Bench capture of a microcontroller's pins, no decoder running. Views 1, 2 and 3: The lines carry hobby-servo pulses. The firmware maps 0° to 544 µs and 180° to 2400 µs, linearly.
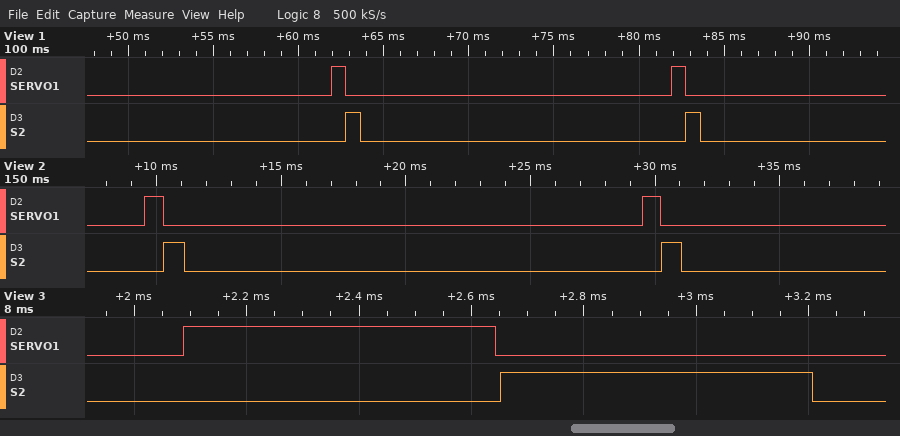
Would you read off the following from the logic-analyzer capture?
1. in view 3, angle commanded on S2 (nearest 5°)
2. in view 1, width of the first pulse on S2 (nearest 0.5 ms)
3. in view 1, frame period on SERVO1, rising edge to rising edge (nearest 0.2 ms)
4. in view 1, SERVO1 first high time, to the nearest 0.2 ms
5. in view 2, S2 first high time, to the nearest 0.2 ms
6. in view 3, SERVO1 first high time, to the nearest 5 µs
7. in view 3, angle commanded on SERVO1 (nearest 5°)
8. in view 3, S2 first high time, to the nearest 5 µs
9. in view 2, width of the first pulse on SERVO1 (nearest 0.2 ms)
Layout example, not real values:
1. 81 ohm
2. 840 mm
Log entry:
1. 0°
2. 1.0 ms
3. 20.0 ms
4. 0.8 ms
5. 0.8 ms
6. 555 µs
7. 0°
8. 555 µs
9. 0.8 ms
